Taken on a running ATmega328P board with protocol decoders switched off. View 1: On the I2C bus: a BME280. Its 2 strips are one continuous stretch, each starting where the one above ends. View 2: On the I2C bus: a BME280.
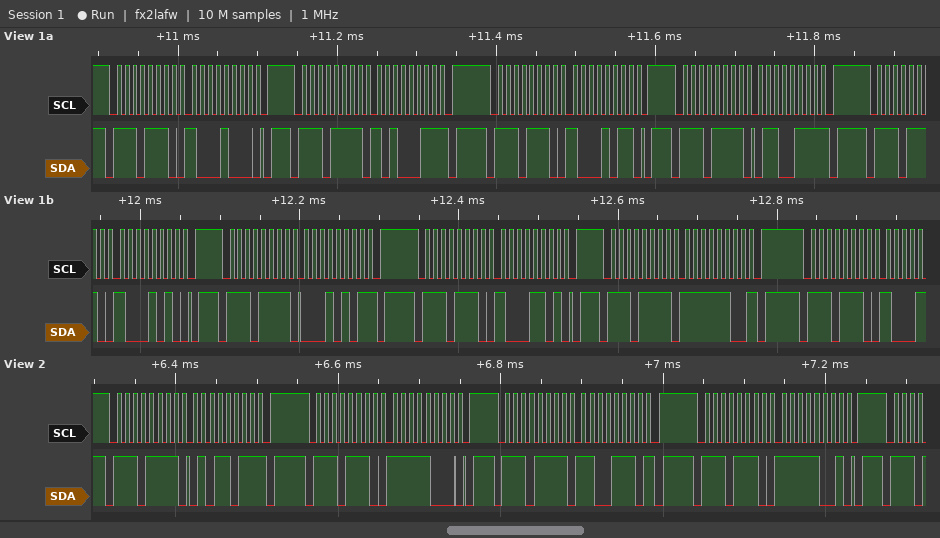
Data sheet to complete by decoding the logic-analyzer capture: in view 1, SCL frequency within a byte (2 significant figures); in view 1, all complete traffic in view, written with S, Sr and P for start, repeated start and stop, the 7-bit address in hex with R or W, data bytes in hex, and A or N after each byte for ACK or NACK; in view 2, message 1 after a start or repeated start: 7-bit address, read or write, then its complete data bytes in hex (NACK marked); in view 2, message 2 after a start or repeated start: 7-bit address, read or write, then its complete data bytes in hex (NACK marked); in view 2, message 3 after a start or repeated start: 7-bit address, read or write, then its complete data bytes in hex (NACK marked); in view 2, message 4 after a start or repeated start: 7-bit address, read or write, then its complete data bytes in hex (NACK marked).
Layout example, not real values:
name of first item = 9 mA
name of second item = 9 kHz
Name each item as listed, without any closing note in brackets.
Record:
in view 1, SCL frequency within a byte = 100 kHz
in view 1, all complete traffic in view, written with S, Sr and P for start, repeated start and stop, the 7-bit address in hex with R or W, data bytes in hex, and A or N after each byte for ACK or NACK = S 77W A 88 A P S 77R A A3 N P S 77W A 8B A P S 77R A 67 N P S 77W A 8A A P S 77R A 15 N P S 77W A 8D A P S 77R A FC N P S 77W A
in view 2, message 1 after a start or repeated start: 7-bit address, read or write, then its complete data bytes in hex = 0x77 read: 5B NACK
in view 2, message 2 after a start or repeated start: 7-bit address, read or write, then its complete data bytes in hex = 0x77 write: F8
in view 2, message 3 after a start or repeated start: 7-bit address, read or write, then its complete data bytes in hex = 0x77 read: CE NACK
in view 2, message 4 after a start or repeated start: 7-bit address, read or write, then its complete data bytes in hex = 0x77 write: F9
